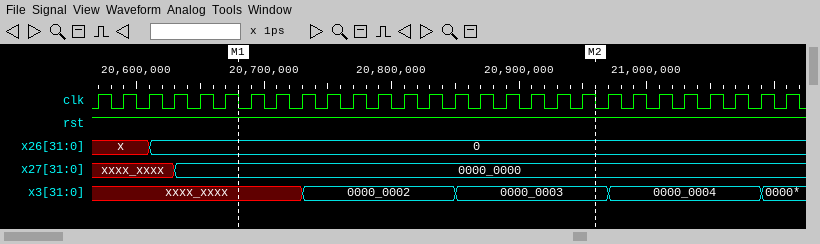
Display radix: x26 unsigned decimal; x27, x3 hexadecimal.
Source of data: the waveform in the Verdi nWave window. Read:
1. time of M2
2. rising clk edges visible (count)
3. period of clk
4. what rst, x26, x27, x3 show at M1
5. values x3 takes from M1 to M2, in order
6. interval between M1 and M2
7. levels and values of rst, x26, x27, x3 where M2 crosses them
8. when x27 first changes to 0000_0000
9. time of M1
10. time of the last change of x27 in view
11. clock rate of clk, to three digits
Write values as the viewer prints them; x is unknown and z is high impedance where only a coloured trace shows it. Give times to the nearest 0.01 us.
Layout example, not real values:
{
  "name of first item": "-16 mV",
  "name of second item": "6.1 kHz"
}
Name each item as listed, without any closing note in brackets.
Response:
{
  "time of M2": "20.96 us",
  "rising clk edges visible": "28",
  "period of clk": "0.02 us",
  "what rst, x26, x27, x3 show at M1": "rst=1, x26=0, x27=0000_0000, x3=xxxx_xxxx",
  "values x3 takes from M1 to M2, in order": "xxxx_xxxx, 0000_0002, 0000_0003",
  "interval between M1 and M2": "0.28 us",
  "levels and values of rst, x26, x27, x3 where M2 crosses them": "rst=1, x26=0, x27=0000_0000, x3=0000_0003",
  "when x27 first changes to 0000_0000": "20.63 us",
  "time of M1": "20.68 us",
  "time of the last change of x27 in view": "20.63 us",
  "clock rate of clk, to three digits": "50.0 MHz"
}
